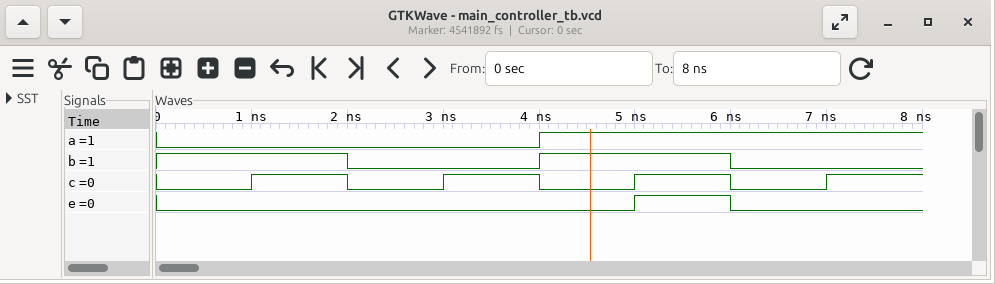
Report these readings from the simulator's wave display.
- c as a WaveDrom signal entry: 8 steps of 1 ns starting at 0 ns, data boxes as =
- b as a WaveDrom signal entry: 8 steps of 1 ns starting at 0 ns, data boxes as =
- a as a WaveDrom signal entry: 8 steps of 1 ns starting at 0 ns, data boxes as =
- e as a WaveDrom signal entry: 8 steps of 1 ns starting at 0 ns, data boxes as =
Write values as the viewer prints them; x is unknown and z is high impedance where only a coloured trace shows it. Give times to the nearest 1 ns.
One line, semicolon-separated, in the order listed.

{name: 'c', wave: '01010101'}; {name: 'b', wave: '1.0.1.0.'}; {name: 'a', wave: '0...1...'}; {name: 'e', wave: '0....10.'}
